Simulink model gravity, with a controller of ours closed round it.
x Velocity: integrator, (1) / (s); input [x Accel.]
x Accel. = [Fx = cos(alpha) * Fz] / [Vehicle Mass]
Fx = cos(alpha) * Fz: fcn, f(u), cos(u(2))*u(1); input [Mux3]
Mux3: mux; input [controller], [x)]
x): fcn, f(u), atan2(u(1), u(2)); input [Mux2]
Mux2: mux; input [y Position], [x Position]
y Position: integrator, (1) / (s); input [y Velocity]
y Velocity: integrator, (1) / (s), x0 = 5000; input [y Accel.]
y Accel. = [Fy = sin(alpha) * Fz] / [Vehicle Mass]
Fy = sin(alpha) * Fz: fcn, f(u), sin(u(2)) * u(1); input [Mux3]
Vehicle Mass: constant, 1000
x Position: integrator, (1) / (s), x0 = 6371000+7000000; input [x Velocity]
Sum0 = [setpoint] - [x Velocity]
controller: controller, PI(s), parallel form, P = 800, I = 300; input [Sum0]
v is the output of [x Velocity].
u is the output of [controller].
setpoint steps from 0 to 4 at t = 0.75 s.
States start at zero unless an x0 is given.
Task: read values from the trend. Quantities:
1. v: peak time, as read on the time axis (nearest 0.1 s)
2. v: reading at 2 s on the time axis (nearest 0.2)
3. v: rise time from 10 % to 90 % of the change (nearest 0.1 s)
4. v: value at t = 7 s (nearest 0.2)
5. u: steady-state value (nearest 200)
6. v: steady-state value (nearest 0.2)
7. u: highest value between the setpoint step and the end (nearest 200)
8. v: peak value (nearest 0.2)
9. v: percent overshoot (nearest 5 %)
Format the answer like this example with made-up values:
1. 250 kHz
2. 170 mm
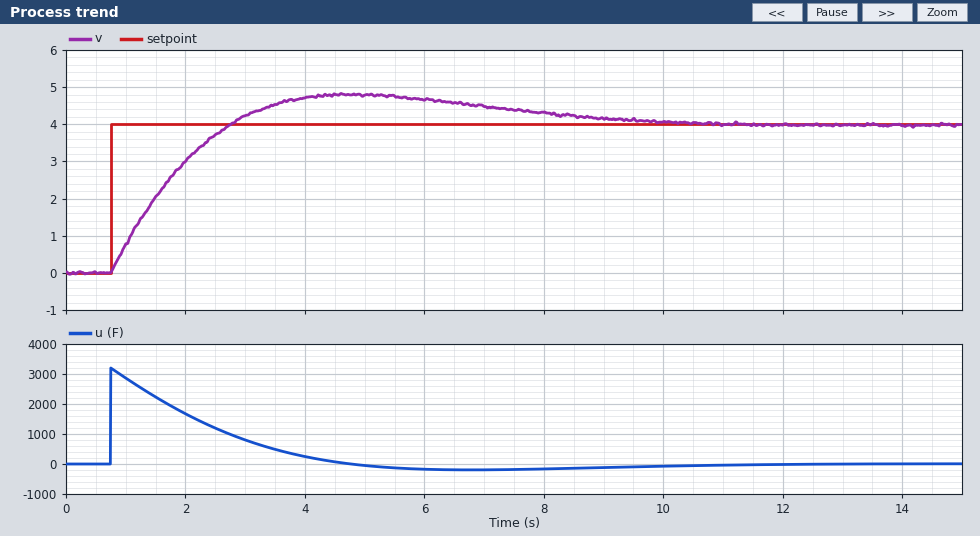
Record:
1. 4.8 s
2. 3.0
3. 1.5 s
4. 4.4
5. 0
6. 4.0
7. 3200
8. 4.8
9. 20 %
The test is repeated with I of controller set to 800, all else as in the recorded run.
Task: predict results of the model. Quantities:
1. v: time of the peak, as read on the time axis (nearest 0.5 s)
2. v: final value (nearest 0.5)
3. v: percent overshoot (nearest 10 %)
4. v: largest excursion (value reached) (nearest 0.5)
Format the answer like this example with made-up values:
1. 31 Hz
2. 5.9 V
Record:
1. 3.5 s
2. 4.0
3. 30 %
4. 5.5
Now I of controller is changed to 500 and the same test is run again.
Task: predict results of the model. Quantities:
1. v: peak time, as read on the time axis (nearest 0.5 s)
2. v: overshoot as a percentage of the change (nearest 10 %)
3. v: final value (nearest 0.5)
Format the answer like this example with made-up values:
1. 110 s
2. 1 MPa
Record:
1. 4.0 s
2. 30 %
3. 4.0
